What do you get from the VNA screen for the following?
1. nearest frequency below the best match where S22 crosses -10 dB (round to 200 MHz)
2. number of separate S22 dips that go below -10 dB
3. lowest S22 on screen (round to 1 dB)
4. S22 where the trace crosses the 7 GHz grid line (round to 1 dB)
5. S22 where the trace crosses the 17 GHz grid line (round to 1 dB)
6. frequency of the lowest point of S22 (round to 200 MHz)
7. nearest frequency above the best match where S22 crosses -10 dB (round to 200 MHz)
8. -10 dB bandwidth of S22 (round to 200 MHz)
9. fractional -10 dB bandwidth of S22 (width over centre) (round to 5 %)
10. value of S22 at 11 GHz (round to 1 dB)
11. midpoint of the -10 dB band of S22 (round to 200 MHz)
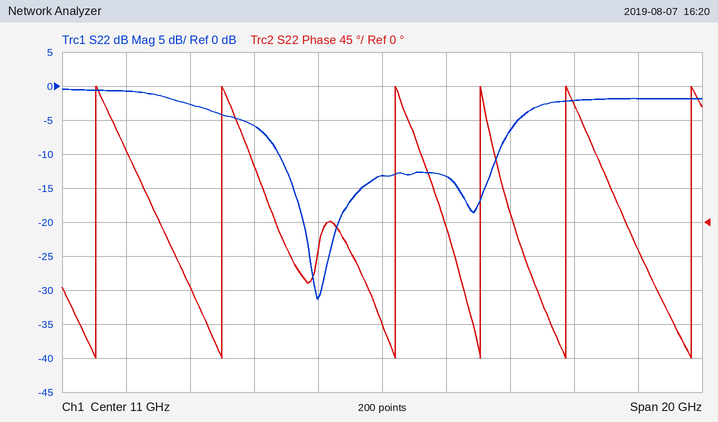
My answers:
7.8 GHz
2
-31 dB
-6 dB
-2 dB
9.0 GHz
14.6 GHz
6.8 GHz
60 %
-13 dB
11.2 GHz
